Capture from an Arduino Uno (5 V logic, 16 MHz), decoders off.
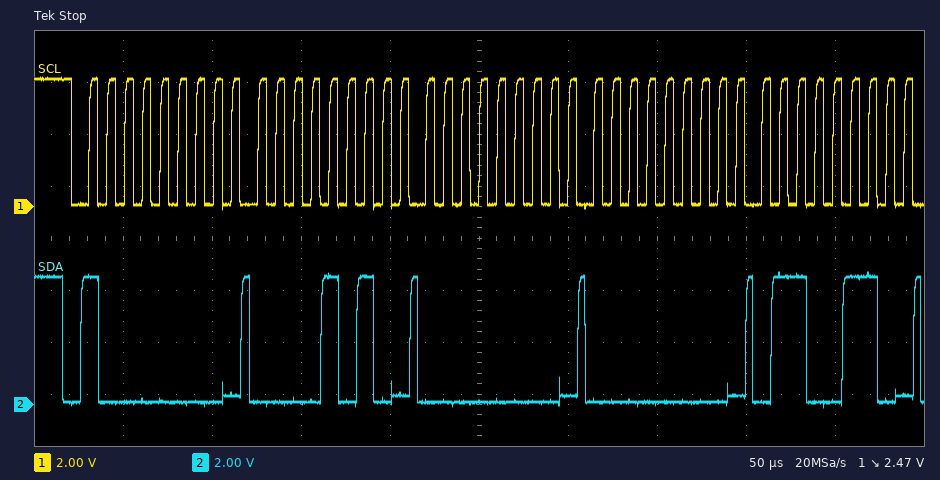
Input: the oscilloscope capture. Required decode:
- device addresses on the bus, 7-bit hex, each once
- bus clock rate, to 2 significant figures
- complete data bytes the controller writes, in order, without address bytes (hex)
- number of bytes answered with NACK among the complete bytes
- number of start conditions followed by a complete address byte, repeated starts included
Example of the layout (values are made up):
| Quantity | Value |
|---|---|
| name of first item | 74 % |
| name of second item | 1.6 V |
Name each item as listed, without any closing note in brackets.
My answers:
| Quantity | Value |
|---|---|
| device addresses on the bus, 7-bit hex, each once | 0x40 |
| bus clock rate, to 2 significant figures | 100 kHz |
| complete data bytes the controller writes, in order, without address bytes | 0A 00 00 66 |
| number of bytes answered with NACK among the complete bytes | 0 |
| number of start conditions followed by a complete address byte, repeated starts included | 1 |
